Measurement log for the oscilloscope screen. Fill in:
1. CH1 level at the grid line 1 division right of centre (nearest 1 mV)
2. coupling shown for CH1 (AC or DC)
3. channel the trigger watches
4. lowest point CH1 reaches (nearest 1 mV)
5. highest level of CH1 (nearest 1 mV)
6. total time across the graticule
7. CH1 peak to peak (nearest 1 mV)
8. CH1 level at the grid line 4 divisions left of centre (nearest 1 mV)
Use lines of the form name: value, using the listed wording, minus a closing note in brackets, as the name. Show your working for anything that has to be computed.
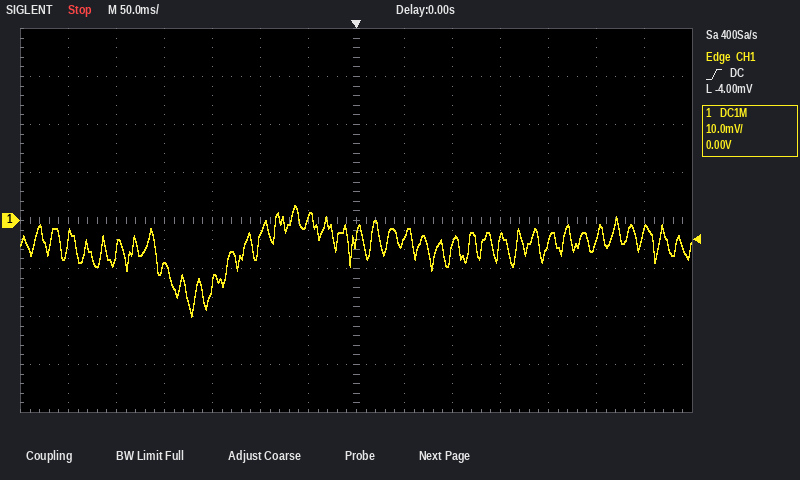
CH1 level at the grid line 1 division right of centre: -4 mV
coupling shown for CH1: DC
channel the trigger watches: CH1
lowest point CH1 reaches: -20 mV
highest level of CH1: 3 mV
total time across the graticule: 700 ms
CH1 peak to peak: 3 mV − (-20 mV) = 23 mV
CH1 level at the grid line 4 divisions left of centre: -9 mV
